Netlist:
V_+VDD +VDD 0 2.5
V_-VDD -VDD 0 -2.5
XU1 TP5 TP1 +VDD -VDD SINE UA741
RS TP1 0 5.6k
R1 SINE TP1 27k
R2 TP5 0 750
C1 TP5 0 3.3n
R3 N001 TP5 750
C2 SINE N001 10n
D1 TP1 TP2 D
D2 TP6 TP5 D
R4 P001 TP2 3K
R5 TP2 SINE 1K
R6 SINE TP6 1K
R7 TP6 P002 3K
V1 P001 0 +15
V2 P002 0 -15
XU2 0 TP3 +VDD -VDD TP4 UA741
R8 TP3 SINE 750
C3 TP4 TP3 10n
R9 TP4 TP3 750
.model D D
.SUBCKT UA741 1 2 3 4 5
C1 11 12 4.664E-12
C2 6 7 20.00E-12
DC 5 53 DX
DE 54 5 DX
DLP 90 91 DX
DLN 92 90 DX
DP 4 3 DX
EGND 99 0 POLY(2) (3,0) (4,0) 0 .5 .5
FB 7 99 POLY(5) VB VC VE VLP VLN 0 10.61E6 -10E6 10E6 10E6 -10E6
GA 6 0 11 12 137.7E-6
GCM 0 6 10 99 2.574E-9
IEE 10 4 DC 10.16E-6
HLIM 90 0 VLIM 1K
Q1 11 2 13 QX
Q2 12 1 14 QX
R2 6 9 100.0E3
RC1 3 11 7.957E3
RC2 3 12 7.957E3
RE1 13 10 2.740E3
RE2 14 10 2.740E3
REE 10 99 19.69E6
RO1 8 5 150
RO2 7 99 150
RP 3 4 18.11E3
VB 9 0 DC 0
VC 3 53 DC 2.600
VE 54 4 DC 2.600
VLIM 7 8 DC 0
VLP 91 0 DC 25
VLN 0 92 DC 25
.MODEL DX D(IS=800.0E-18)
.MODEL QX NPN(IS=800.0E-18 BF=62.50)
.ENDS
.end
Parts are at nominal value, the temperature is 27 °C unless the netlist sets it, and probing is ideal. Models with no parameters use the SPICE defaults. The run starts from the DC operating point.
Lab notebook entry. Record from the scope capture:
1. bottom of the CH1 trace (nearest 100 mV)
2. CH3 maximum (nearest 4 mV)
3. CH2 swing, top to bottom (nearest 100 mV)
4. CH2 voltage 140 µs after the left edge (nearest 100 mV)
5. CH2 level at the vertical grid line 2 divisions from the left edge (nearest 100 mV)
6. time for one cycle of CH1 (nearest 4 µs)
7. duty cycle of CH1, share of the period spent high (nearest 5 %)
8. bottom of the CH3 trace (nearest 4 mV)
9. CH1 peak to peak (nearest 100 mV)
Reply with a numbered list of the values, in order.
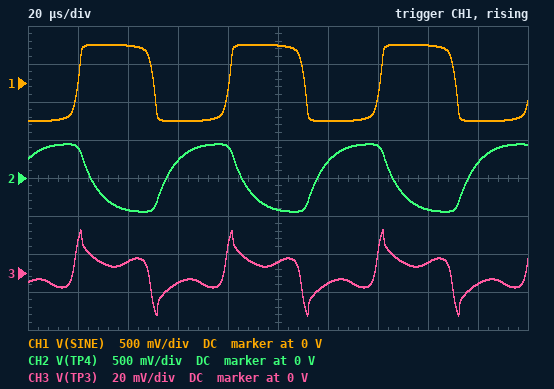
1. -500 mV
2. 24 mV
3. 900 mV
4. 400 mV
5. -400 mV
6. 60 µs
7. 50 %
8. -24 mV
9. 1.0 V
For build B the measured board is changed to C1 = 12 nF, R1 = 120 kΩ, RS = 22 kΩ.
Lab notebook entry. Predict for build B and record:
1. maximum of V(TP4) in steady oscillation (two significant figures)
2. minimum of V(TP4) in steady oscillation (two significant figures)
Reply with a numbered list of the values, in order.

1. 450 mV
2. -450 mV
